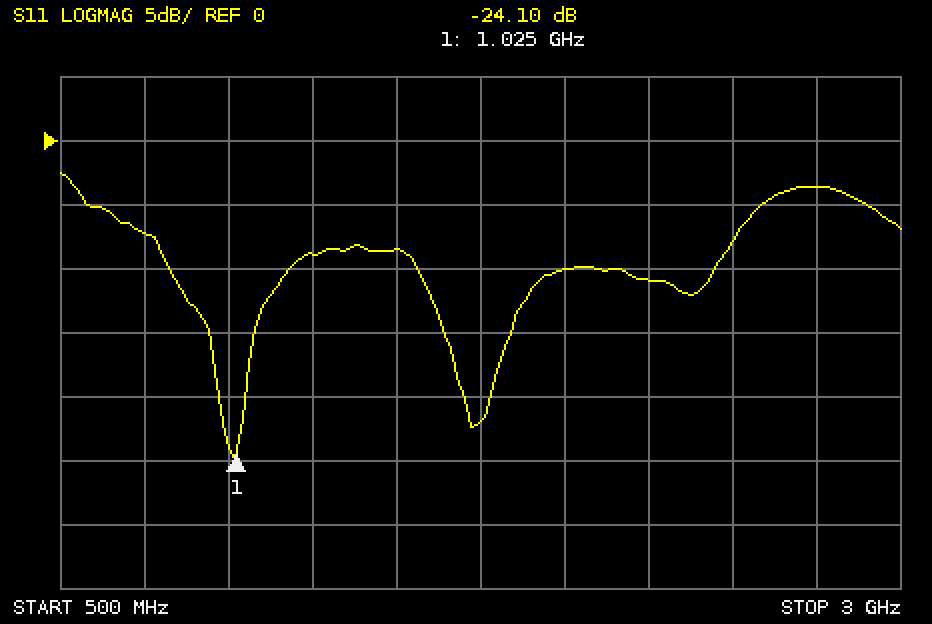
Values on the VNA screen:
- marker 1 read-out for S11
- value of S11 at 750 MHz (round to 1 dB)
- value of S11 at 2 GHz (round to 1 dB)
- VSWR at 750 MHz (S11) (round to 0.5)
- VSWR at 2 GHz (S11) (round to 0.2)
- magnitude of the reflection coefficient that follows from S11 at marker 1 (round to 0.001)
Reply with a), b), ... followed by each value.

a) -24.10 dB
b) -7 dB
c) -10 dB
d) 2.5
e) 2.0
f) 0.062
